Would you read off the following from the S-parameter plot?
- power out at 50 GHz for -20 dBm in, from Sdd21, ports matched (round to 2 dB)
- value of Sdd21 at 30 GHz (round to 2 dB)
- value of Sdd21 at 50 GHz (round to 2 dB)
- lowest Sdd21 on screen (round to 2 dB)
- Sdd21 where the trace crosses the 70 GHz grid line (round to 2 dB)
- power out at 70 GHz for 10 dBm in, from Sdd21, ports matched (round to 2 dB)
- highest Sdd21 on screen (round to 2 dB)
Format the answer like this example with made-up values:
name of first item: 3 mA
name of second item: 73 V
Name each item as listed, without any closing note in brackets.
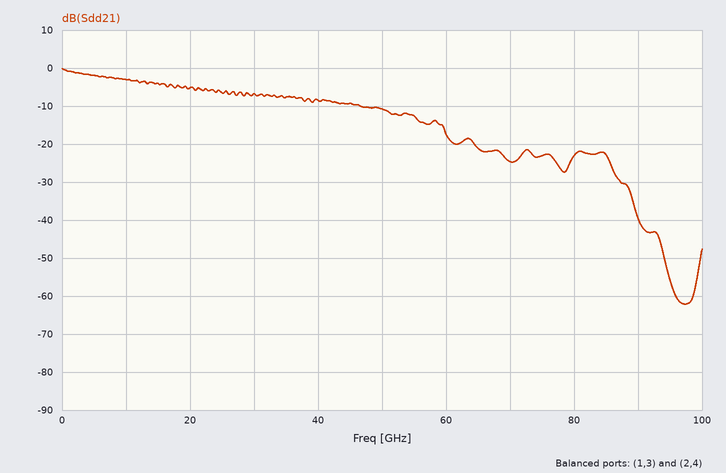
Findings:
power out at 50 GHz for -20 dBm in, from Sdd21, ports matched: -30 dBm
value of Sdd21 at 30 GHz: -6 dB
value of Sdd21 at 50 GHz: -10 dB
lowest Sdd21 on screen: -62 dB
Sdd21 where the trace crosses the 70 GHz grid line: -24 dB
power out at 70 GHz for 10 dBm in, from Sdd21, ports matched: -14 dBm
highest Sdd21 on screen: 0 dB
